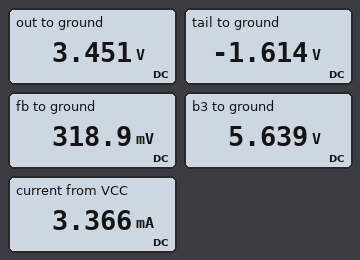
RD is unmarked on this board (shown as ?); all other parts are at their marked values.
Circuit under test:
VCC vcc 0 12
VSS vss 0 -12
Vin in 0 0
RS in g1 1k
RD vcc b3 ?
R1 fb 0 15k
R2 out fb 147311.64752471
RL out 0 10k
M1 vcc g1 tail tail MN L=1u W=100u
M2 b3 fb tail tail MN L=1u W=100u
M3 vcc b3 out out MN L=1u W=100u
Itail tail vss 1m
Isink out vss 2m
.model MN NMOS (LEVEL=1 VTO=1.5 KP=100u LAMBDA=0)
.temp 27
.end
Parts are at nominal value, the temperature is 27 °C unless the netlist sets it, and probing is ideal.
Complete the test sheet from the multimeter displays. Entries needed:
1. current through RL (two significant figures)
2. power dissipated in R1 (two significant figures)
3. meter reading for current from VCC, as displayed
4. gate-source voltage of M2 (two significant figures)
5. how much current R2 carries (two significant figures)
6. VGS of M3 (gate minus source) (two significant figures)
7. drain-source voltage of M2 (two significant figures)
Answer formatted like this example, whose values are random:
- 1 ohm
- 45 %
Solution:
- 350 µA
- 6.8 µW
- 3.366 mA
- 1.9 V
- 21 µA
- 2.2 V
- 7.3 V
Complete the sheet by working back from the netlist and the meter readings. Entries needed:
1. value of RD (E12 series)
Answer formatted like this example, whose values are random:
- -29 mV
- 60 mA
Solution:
- 6.8 kΩ
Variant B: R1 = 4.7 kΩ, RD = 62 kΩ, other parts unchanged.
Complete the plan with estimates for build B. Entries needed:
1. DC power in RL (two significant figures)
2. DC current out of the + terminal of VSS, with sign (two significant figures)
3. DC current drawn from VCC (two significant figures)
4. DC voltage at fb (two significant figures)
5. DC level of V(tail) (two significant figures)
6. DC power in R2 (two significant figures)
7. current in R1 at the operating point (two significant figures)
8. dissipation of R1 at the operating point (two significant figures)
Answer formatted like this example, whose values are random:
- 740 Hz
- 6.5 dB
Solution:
- 1.5 mW
- -3.0 mA
- 2.6 mA
- -120 mV
- -1.9 V
- 95 µW
- 25 µA
- 3.0 µW
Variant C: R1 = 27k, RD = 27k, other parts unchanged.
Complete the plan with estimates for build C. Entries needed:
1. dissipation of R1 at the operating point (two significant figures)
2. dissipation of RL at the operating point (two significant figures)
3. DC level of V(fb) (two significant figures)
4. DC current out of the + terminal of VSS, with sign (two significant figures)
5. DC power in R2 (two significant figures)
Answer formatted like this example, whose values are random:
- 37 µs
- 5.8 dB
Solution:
- 200 nW
- 23 µW
- -74 mV
- -3.0 mA
- 1.1 µW
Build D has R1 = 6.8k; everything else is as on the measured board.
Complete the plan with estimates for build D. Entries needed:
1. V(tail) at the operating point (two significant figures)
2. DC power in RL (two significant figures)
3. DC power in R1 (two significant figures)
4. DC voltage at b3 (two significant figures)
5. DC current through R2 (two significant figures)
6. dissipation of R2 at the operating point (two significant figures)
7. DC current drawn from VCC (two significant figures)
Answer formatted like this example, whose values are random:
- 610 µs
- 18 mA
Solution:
- -1.7 V
- 1.9 mW
- 5.6 µW
- 6.6 V
- 29 µA
- 120 µW
- 3.5 mA
